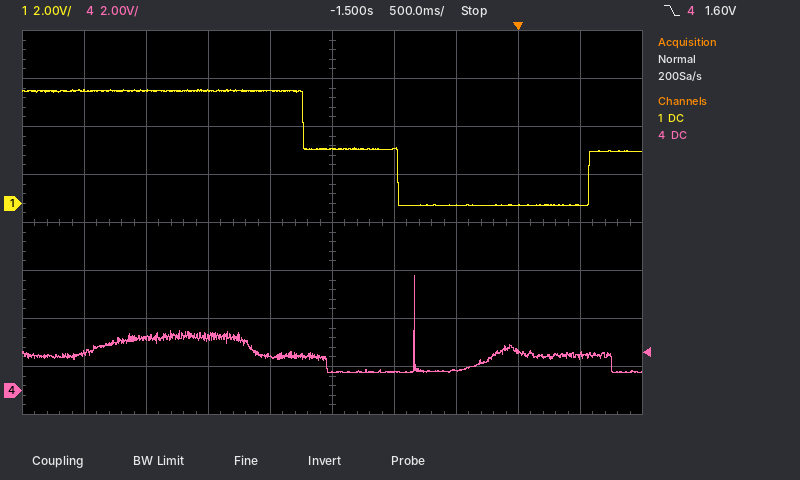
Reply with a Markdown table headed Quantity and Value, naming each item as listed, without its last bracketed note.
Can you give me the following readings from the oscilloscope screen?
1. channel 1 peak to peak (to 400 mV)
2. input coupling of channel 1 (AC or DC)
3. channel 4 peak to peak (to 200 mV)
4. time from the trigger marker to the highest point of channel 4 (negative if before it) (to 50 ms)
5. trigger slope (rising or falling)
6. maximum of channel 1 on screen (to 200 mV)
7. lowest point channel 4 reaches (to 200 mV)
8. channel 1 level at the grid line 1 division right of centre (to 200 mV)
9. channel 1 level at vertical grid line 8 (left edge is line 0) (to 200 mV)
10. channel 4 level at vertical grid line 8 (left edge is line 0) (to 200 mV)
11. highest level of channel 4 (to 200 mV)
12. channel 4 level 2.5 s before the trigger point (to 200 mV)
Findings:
| Quantity | Value |
|---|---|
| channel 1 peak to peak | 4.8 V |
| input coupling of channel 1 | DC |
| channel 4 peak to peak | 4.0 V |
| time from the trigger marker to the highest point of channel 4 (negative if before it) | -850 ms |
| trigger slope | falling |
| maximum of channel 1 on screen | 4.8 V |
| lowest point channel 4 reaches | 800 mV |
| channel 1 level at the grid line 1 division right of centre | 2.2 V |
| channel 1 level at vertical grid line 8 (left edge is line 0) | 0.0 V |
| channel 4 level at vertical grid line 8 (left edge is line 0) | 1.6 V |
| highest level of channel 4 | 4.8 V |
| channel 4 level 2.5 s before the trigger point | 2.2 V |
